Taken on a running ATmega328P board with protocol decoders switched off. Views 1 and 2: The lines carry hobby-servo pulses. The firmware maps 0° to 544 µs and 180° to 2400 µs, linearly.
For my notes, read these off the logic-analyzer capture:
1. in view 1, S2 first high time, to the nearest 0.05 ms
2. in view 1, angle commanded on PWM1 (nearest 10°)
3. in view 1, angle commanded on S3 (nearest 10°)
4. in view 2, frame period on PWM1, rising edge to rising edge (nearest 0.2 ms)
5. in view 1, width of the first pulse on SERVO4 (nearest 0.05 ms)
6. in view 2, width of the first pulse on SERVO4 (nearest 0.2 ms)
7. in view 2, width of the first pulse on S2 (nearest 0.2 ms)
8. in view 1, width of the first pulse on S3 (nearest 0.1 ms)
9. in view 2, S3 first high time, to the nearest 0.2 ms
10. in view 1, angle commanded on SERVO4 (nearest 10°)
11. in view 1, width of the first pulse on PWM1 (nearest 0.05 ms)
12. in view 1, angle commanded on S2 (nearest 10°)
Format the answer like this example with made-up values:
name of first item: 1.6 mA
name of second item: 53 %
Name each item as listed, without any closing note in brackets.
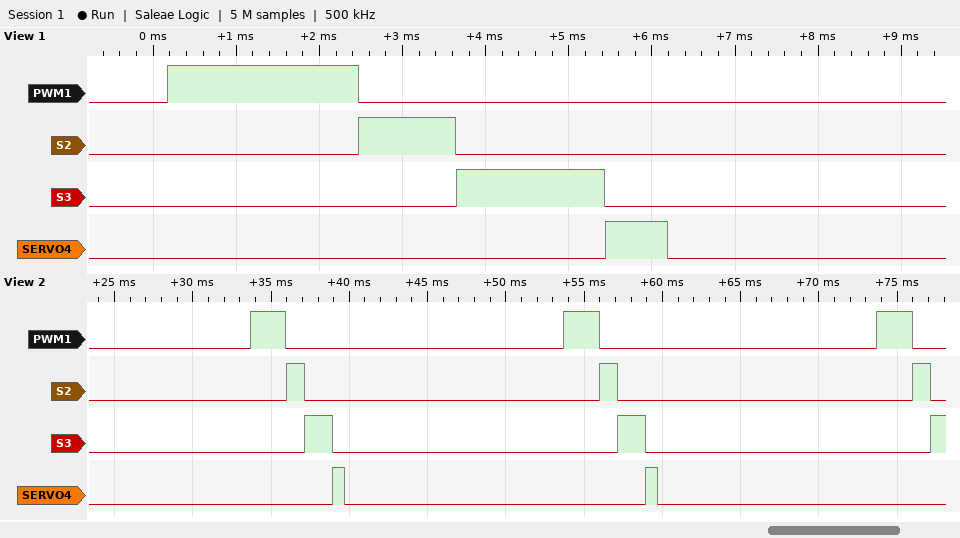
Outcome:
in view 1, S2 first high time, to the nearest 0.05 ms: 1.15 ms
in view 1, angle commanded on PWM1: 170°
in view 1, angle commanded on S3: 120°
in view 2, frame period on PWM1, rising edge to rising edge: 20.0 ms
in view 1, width of the first pulse on SERVO4: 0.75 ms
in view 2, width of the first pulse on SERVO4: 0.8 ms
in view 2, width of the first pulse on S2: 1.2 ms
in view 1, width of the first pulse on S3: 1.8 ms
in view 2, S3 first high time, to the nearest 0.2 ms: 1.8 ms
in view 1, angle commanded on SERVO4: 20°
in view 1, width of the first pulse on PWM1: 2.30 ms
in view 1, angle commanded on S2: 60°
